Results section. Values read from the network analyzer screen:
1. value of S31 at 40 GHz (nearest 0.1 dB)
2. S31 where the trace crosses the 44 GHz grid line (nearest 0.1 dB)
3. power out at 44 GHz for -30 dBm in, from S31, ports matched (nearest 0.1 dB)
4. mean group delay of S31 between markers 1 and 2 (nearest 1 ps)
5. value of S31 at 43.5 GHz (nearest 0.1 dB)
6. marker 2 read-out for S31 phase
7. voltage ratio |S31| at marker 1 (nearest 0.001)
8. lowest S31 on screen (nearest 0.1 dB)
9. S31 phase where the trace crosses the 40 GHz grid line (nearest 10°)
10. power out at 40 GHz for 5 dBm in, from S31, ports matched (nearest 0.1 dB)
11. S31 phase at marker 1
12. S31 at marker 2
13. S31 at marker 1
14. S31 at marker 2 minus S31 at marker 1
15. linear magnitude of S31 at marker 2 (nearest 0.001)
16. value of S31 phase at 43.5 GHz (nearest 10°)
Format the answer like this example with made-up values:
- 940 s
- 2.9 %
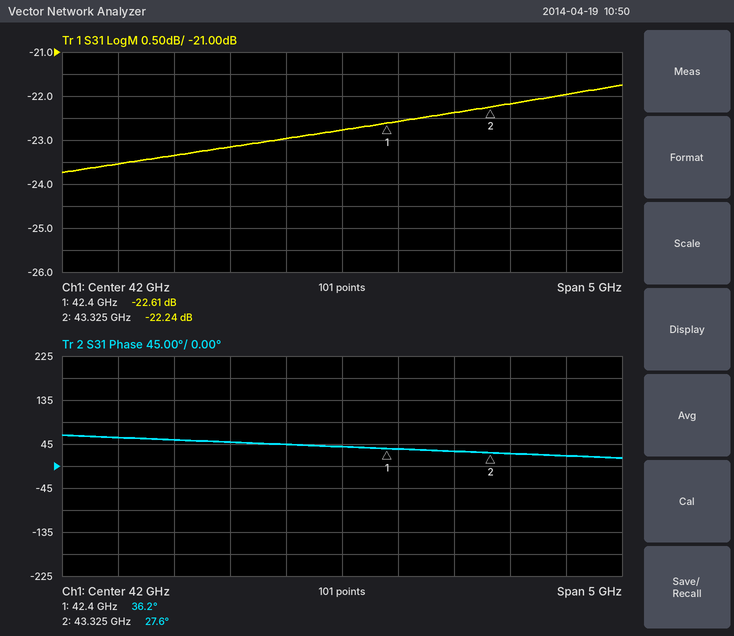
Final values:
- -23.5 dB
- -22.0 dB
- -52.0 dBm
- 26 ps
- -22.2 dB
- 27.6°
- 0.074
- -23.7 dB
- 60°
- -18.5 dBm
- 36.2°
- -22.24 dB
- -22.61 dB
- 0.37 dB
- 0.077
- 30°
